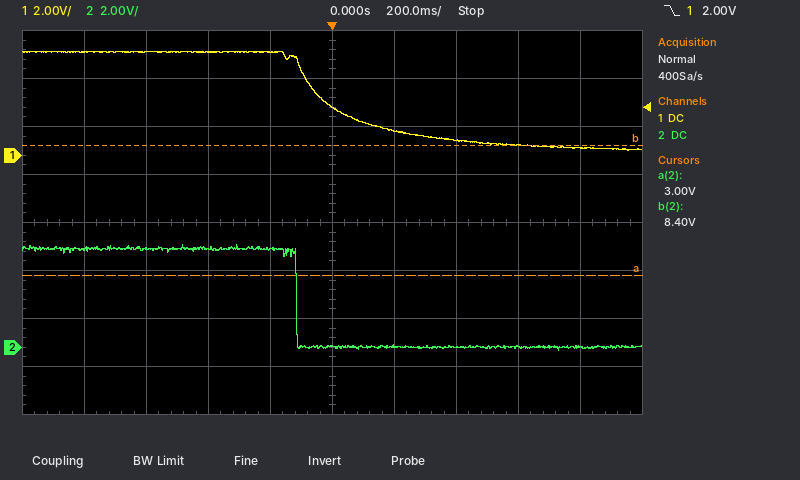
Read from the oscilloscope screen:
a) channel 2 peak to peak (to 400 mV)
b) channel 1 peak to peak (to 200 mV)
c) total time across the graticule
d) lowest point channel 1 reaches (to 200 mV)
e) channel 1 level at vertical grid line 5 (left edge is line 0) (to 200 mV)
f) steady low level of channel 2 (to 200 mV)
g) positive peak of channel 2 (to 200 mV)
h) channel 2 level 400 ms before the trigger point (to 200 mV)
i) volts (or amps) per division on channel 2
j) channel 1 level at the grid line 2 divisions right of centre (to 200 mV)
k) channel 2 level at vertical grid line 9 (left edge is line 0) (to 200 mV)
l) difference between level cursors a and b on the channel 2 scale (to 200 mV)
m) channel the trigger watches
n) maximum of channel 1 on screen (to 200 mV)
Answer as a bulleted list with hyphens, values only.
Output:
- 4.4 V
- 4.2 V
- 2 s
- 200 mV
- 2.0 V
- 0.0 V
- 4.2 V
- 4.2 V
- 2 V
- 600 mV
- 0.0 V
- 5.4 V
- channel 1
- 4.4 V
